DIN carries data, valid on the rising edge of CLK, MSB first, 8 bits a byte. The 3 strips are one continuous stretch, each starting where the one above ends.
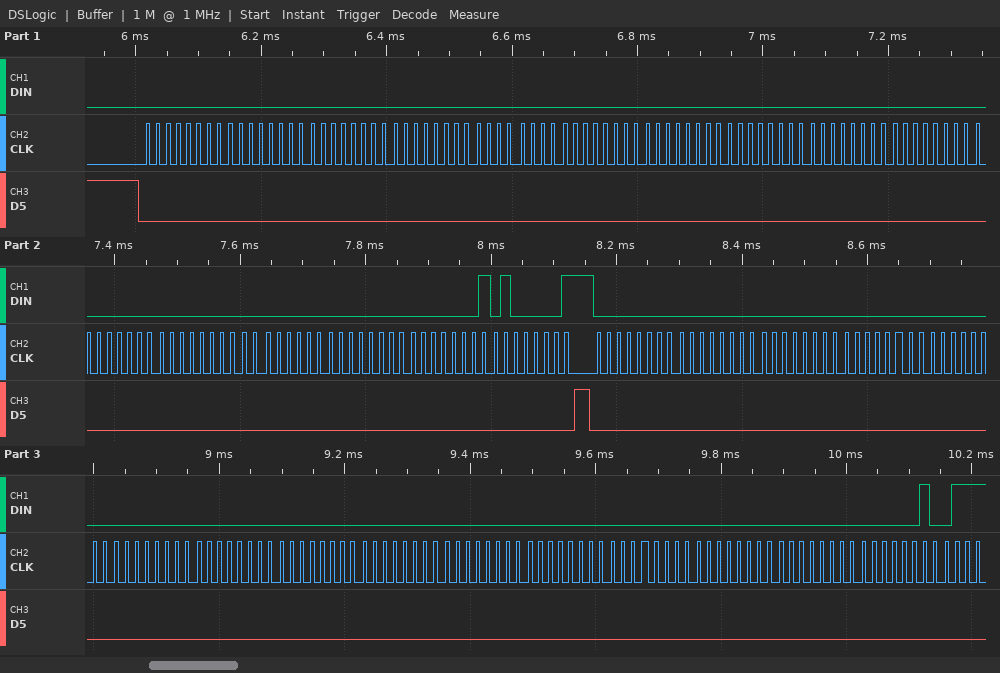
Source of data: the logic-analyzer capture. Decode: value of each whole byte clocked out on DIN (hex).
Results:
00 00 00 00 00 00 00 00 00 00 00 00 00 00 01 41 00 00 00 00 00 00 00 00 00 00 00 00 00 00 02
